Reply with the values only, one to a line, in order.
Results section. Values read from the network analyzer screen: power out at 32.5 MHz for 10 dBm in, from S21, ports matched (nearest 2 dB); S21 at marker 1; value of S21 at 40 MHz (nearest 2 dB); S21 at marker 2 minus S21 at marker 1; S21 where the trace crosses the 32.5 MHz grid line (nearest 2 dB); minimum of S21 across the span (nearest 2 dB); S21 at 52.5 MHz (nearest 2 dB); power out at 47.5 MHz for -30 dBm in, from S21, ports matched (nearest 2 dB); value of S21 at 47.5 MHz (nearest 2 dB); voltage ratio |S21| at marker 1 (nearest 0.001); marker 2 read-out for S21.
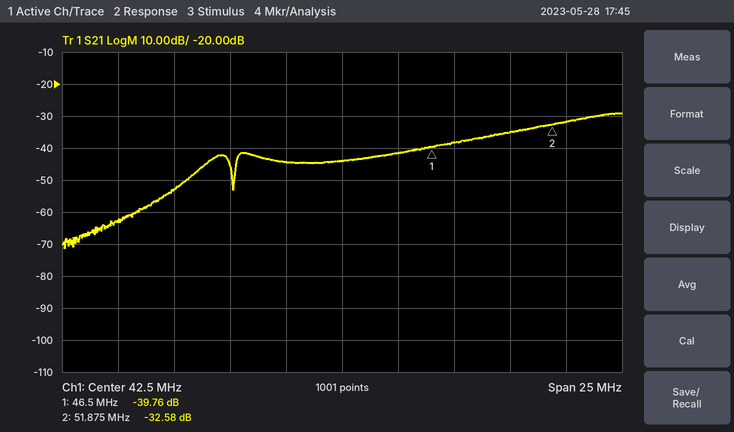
-52 dBm
-39.76 dB
-44 dB
7.18 dB
-62 dB
-72 dB
-32 dB
-68 dBm
-38 dB
0.010
-32.58 dB
